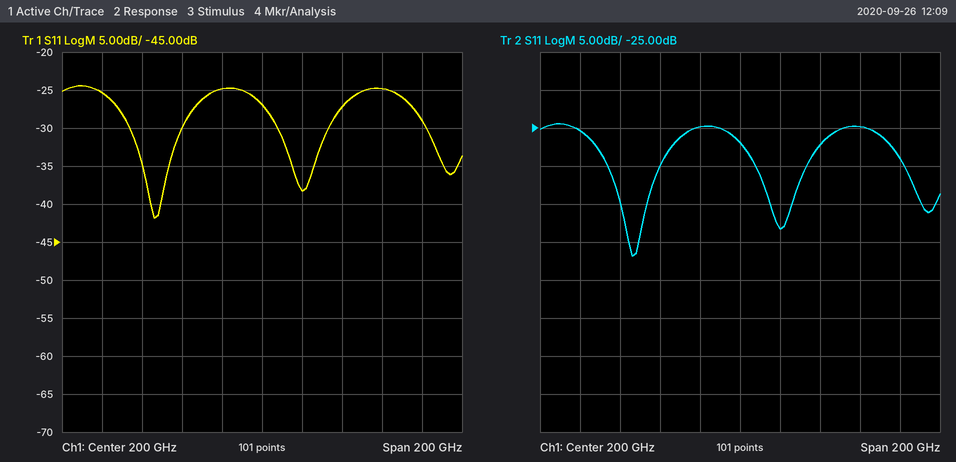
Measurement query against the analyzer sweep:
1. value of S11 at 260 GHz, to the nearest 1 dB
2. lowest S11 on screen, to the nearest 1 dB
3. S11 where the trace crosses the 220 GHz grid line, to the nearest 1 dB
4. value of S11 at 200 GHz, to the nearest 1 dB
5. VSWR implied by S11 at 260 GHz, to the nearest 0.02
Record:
-25 dB
-42 dB
-38 dB
-27 dB
1.12
